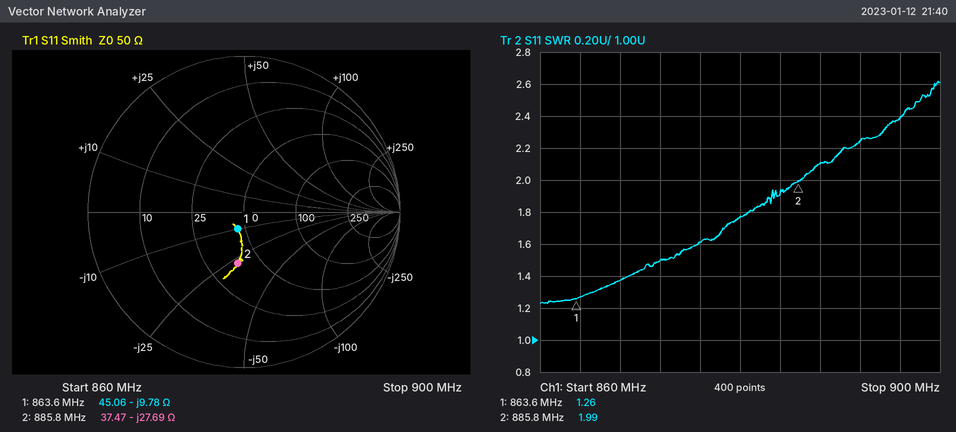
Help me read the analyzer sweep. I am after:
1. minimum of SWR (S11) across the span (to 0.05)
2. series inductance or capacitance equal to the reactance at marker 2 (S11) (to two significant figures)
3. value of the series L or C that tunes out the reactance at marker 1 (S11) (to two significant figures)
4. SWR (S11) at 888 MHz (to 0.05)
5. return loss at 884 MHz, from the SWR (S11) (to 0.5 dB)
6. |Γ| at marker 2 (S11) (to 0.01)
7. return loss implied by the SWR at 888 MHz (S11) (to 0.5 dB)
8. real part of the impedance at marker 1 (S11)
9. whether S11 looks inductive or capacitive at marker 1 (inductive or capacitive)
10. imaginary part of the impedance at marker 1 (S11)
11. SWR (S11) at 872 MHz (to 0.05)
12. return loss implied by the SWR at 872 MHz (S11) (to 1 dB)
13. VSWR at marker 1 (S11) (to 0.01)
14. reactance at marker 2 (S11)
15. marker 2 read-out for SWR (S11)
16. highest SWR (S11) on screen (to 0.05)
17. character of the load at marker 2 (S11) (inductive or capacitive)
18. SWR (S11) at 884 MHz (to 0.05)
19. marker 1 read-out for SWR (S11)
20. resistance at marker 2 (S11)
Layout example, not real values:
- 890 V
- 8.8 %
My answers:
- 1.25
- 6.5 pF
- 1.8 nH
- 2.10
- 10.0 dB
- 0.33
- 9.0 dB
- 45.06 Ω
- capacitive
- -9.78 Ω
- 1.50
- 14 dB
- 1.26
- -27.69 Ω
- 1.99
- 2.60
- capacitive
- 1.90
- 1.26
- 37.47 Ω
